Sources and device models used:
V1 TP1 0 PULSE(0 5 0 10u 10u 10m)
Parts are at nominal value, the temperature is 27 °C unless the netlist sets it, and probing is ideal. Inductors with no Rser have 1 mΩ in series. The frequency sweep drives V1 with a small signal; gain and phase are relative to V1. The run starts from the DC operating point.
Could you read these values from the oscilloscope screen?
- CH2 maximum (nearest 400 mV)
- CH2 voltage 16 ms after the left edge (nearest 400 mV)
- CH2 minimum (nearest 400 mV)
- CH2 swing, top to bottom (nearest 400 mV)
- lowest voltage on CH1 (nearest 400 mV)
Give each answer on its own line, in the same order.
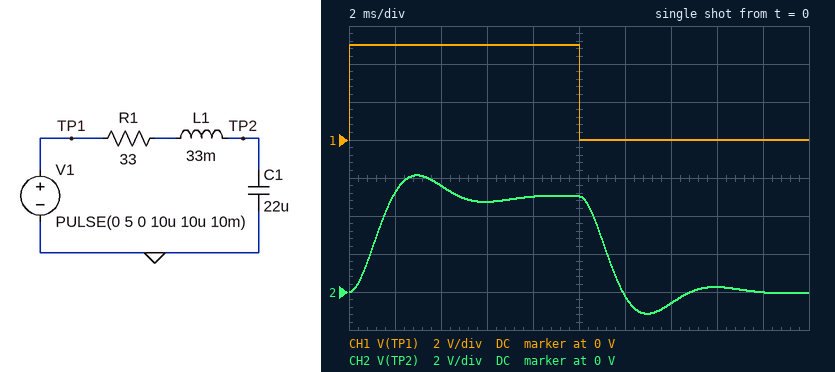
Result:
6.0 V
400 mV
-1.2 V
7.2 V
0 V
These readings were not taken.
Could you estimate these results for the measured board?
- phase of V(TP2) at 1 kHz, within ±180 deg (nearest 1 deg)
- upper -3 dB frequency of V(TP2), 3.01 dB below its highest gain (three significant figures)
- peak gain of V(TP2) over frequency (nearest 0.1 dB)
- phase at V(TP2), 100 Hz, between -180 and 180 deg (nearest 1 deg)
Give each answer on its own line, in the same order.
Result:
-171 deg
222 Hz
2.3 dB
-33 deg
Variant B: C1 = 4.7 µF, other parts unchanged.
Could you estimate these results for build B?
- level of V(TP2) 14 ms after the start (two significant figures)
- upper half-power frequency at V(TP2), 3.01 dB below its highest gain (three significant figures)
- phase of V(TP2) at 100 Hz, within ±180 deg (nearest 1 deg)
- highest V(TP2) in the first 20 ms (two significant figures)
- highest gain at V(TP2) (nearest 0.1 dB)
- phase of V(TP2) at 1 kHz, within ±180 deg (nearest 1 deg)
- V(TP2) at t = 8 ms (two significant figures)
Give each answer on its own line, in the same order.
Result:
-660 mV
462 Hz
-6 deg
7.7 V
8.3 dB
-169 deg
4.9 V
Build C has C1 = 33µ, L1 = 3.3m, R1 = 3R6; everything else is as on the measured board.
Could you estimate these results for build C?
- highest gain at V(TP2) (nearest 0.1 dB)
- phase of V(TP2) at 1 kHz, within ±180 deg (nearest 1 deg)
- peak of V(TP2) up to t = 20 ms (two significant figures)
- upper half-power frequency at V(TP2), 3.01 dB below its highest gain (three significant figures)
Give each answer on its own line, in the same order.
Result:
9.0 dB
-167 deg
7.8 V
548 Hz
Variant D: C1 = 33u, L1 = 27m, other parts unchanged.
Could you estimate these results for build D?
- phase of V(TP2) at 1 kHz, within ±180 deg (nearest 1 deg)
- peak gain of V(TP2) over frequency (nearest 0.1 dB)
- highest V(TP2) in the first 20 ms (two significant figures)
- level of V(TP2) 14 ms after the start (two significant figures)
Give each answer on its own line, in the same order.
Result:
-169 deg
0.5 dB
5.5 V
-510 mV
